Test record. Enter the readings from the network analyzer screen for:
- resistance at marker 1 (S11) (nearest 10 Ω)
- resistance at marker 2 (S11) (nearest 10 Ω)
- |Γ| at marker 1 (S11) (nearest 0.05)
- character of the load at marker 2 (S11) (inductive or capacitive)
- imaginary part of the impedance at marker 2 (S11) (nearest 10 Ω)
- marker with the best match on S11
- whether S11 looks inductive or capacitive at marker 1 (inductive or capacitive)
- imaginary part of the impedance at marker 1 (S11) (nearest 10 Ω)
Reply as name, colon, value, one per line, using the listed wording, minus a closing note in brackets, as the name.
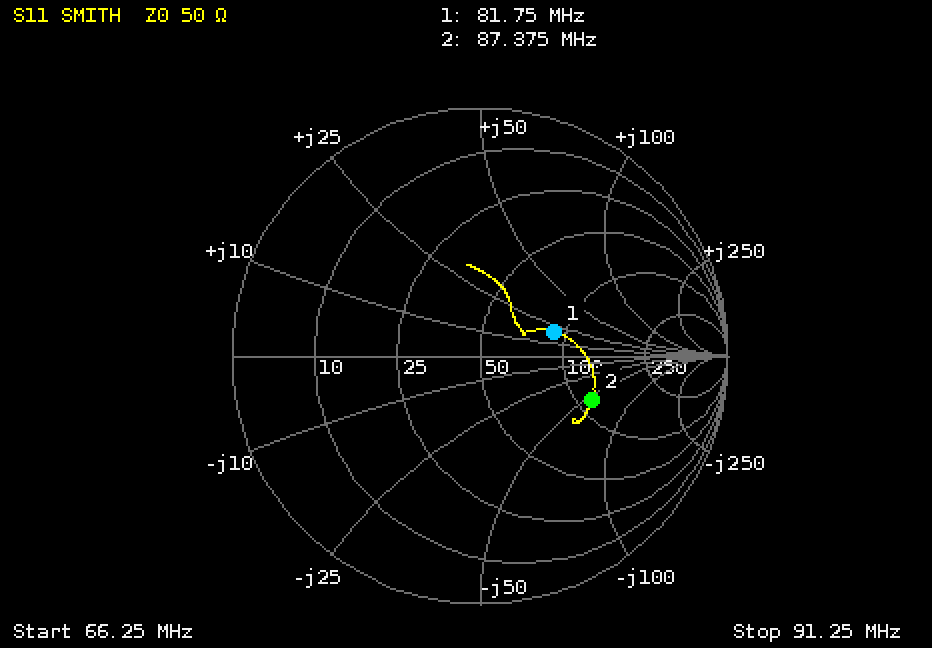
resistance at marker 1 (S11): 90 Ω
resistance at marker 2 (S11): 110 Ω
|Γ| at marker 1 (S11): 0.30
character of the load at marker 2 (S11): capacitive
imaginary part of the impedance at marker 2 (S11): -50 Ω
marker with the best match on S11: marker 1
whether S11 looks inductive or capacitive at marker 1: inductive
imaginary part of the impedance at marker 1 (S11): +20 Ω
